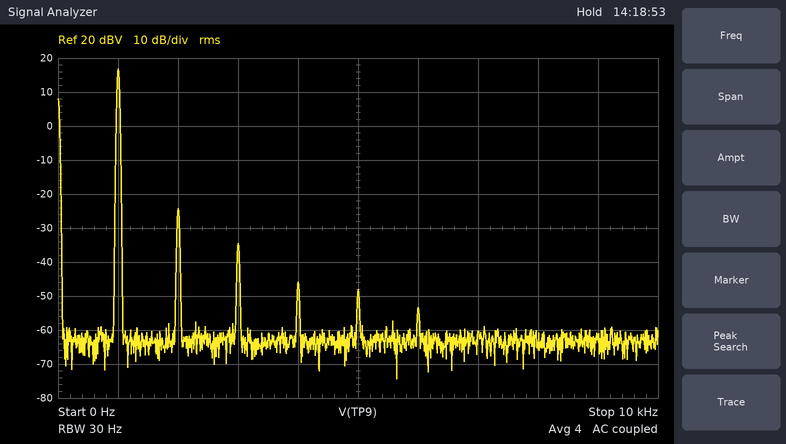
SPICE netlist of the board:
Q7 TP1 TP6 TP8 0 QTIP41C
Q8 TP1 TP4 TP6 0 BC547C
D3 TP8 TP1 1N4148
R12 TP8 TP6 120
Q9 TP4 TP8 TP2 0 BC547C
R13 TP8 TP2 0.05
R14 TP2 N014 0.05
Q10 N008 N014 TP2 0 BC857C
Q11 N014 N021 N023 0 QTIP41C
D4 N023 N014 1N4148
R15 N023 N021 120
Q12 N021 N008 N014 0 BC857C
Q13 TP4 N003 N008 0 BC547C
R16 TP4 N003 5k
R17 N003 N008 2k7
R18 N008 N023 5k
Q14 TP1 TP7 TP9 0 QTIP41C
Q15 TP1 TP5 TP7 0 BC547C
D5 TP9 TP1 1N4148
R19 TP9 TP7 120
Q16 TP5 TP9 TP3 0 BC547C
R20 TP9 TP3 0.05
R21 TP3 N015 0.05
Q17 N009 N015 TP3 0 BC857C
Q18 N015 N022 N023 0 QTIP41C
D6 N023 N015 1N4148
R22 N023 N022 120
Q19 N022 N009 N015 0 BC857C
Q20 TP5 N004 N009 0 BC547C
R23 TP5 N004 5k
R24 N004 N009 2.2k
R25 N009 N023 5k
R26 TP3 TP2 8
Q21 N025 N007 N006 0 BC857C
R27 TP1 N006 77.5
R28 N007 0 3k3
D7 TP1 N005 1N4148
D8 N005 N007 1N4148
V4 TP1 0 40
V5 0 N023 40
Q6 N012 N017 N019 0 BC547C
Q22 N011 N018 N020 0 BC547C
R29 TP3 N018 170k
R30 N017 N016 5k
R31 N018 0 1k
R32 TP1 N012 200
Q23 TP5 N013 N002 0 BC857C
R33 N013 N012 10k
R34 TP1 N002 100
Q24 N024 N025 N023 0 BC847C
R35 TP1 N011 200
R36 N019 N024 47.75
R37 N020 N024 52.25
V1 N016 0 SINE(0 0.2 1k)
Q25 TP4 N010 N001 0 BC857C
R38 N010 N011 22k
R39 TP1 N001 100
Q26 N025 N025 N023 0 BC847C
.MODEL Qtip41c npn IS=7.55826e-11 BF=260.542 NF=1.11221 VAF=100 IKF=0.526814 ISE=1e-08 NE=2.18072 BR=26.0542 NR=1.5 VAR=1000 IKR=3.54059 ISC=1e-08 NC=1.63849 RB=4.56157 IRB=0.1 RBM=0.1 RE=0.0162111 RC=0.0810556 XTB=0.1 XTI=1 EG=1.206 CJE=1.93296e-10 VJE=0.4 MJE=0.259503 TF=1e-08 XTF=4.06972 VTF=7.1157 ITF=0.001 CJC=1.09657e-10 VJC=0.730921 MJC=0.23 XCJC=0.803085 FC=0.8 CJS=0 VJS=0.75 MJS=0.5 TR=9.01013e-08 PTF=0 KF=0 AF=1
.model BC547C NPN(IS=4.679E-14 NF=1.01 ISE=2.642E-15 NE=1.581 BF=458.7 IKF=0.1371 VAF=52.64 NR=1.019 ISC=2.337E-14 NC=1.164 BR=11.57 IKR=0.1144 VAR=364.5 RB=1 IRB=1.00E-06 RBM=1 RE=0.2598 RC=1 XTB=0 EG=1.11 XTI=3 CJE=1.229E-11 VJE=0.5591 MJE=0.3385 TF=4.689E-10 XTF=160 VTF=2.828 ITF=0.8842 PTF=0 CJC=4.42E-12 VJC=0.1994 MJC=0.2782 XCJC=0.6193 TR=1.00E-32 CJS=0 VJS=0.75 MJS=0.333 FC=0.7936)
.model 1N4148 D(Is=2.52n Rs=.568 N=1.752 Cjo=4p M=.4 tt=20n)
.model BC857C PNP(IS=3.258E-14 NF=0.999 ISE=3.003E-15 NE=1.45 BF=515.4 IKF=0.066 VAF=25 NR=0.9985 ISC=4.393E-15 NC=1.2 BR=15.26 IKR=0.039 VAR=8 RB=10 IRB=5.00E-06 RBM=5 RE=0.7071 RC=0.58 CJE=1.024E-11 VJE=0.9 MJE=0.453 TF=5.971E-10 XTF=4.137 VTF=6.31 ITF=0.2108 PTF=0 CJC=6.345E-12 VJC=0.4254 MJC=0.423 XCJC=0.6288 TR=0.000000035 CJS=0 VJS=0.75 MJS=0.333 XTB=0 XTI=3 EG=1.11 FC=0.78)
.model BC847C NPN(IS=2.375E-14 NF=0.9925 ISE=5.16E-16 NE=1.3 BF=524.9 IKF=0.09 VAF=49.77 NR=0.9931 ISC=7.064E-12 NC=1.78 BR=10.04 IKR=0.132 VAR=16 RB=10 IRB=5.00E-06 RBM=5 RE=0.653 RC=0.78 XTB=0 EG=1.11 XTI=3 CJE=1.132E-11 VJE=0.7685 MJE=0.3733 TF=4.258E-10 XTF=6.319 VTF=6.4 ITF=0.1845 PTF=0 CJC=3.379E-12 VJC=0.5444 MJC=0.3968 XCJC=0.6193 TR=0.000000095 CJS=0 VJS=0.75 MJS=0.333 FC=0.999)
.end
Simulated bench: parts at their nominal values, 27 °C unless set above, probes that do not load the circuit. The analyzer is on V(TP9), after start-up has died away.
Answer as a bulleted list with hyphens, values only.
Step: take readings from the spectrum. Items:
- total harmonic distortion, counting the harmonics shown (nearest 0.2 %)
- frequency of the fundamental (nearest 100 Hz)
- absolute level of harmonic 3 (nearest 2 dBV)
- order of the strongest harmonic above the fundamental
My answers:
- 1.0 %
- 1.0 kHz
- -34 dBV
- 2
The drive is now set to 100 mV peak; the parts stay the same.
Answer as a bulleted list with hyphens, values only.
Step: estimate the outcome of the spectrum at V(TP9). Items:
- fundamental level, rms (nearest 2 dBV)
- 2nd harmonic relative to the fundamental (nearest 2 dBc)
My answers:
- 10 dBV
- -48 dBc
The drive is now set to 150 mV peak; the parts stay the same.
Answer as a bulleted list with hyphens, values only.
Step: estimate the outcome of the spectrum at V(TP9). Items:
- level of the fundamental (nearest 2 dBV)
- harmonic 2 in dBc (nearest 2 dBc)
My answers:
- 14 dBV
- -44 dBc
